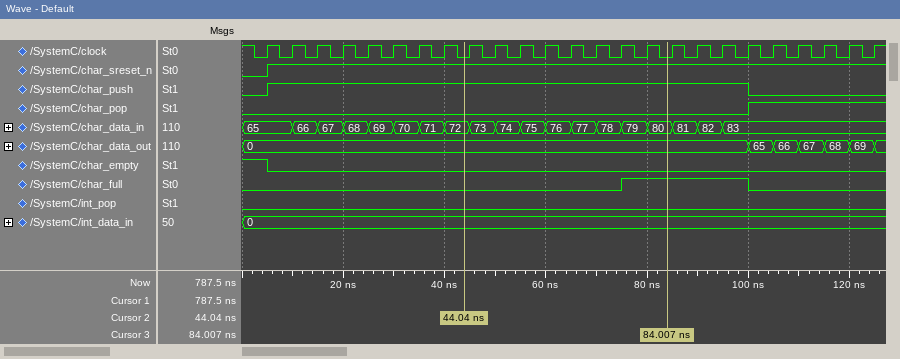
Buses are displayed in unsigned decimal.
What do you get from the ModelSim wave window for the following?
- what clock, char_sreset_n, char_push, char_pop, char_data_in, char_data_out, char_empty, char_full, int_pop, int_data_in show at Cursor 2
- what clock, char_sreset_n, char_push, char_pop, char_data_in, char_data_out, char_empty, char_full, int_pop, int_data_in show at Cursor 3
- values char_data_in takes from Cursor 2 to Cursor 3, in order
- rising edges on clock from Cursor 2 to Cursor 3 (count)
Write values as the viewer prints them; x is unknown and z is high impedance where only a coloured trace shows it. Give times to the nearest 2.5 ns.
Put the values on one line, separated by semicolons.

clock=0, char_sreset_n=1, char_push=1, char_pop=0, char_data_in=72, char_data_out=0, char_empty=0, char_full=0, int_pop=0, int_data_in=0; clock=0, char_sreset_n=1, char_push=1, char_pop=0, char_data_in=80, char_data_out=0, char_empty=0, char_full=1, int_pop=0, int_data_in=0; 72, 73, 74, 75, 76, 77, 78, 79, 80; 8
